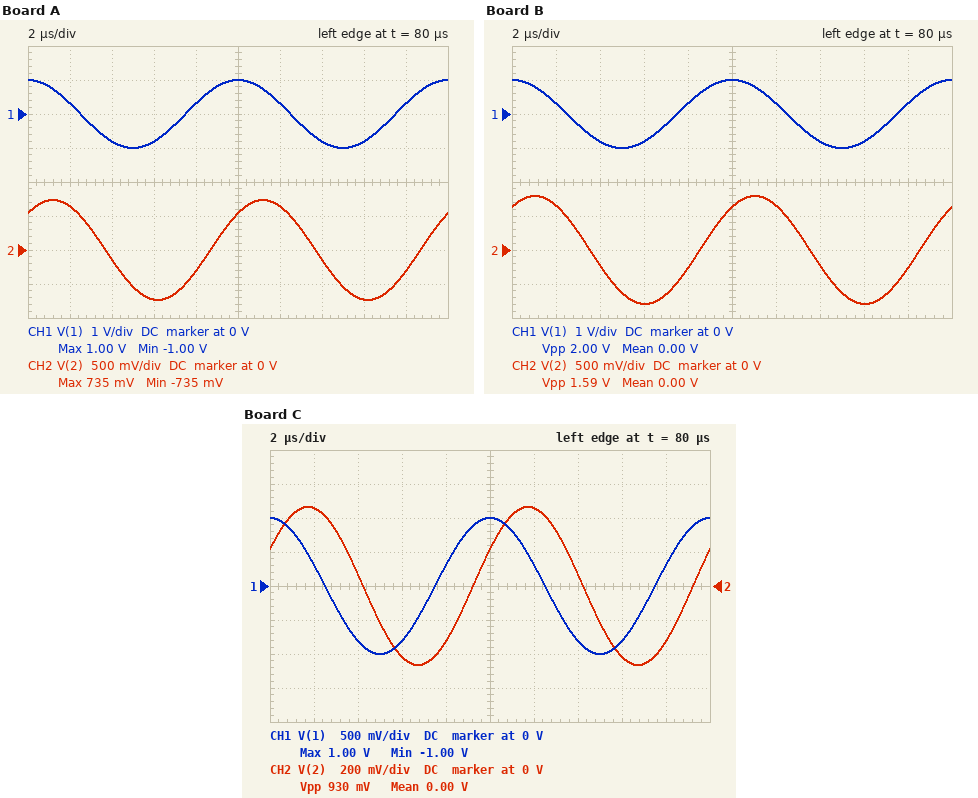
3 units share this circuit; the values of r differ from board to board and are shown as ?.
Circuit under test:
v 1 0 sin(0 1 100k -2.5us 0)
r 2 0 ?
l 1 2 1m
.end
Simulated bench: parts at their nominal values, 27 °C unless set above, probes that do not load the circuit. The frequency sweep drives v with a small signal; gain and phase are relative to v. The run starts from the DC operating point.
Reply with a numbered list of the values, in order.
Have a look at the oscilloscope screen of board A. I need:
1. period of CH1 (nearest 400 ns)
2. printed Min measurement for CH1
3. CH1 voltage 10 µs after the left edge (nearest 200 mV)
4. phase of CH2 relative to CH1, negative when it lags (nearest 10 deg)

1. 10.0 µs
2. -1.00 V
3. 1.0 V
4. -40 deg
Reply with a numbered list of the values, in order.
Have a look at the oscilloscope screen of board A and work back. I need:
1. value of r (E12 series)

1. 680 Ω
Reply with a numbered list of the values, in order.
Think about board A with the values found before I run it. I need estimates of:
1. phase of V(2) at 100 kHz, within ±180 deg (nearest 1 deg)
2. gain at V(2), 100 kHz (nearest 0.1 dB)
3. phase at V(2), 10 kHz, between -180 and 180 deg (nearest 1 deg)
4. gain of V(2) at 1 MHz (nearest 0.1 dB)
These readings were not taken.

1. -43 deg
2. -2.7 dB
3. -5 deg
4. -19.4 dB
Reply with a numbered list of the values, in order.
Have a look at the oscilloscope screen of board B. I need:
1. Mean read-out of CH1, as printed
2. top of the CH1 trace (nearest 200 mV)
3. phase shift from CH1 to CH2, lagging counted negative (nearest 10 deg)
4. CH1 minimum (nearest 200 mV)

1. 0.00 V
2. 1.0 V
3. -40 deg
4. -1.0 V
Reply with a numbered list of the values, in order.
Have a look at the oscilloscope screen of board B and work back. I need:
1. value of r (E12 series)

1. 820 Ω
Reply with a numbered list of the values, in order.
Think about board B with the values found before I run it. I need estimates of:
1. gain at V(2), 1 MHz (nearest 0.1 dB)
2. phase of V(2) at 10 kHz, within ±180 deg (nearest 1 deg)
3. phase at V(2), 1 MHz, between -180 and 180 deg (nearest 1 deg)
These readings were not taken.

1. -17.8 dB
2. -4 deg
3. -83 deg
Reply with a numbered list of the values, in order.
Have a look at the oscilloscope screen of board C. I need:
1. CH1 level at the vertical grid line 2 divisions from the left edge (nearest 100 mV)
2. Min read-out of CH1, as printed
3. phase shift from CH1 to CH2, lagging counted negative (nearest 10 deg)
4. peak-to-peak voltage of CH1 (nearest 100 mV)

1. -800 mV
2. -1.00 V
3. -60 deg
4. 2.0 V
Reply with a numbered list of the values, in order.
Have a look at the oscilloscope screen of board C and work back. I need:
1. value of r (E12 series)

1. 330 Ω
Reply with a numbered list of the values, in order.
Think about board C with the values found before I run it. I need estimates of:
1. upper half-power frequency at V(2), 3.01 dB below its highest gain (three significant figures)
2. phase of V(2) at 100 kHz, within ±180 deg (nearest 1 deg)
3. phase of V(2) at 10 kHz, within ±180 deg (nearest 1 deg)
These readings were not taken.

1. 52.5 kHz
2. -62 deg
3. -11 deg
